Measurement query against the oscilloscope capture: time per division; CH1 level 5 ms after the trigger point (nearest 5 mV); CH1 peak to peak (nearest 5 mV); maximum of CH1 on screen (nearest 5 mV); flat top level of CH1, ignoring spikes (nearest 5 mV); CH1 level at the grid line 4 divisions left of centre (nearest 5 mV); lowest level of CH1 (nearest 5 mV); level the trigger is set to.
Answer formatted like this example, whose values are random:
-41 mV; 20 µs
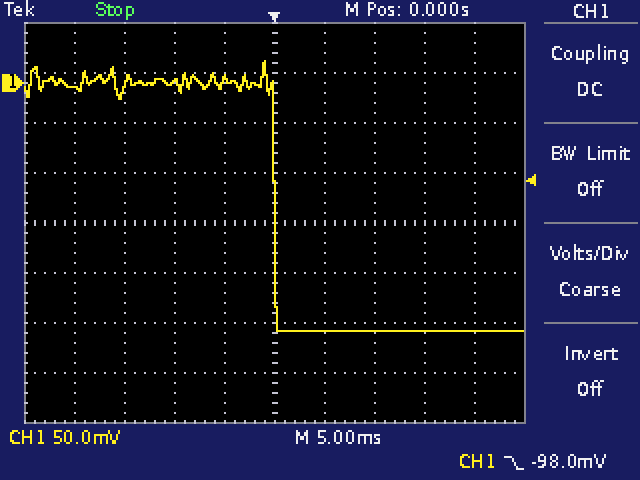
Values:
5 ms; -250 mV; 270 mV; 20 mV; 0 mV; -5 mV; -250 mV; -98.0 mV
